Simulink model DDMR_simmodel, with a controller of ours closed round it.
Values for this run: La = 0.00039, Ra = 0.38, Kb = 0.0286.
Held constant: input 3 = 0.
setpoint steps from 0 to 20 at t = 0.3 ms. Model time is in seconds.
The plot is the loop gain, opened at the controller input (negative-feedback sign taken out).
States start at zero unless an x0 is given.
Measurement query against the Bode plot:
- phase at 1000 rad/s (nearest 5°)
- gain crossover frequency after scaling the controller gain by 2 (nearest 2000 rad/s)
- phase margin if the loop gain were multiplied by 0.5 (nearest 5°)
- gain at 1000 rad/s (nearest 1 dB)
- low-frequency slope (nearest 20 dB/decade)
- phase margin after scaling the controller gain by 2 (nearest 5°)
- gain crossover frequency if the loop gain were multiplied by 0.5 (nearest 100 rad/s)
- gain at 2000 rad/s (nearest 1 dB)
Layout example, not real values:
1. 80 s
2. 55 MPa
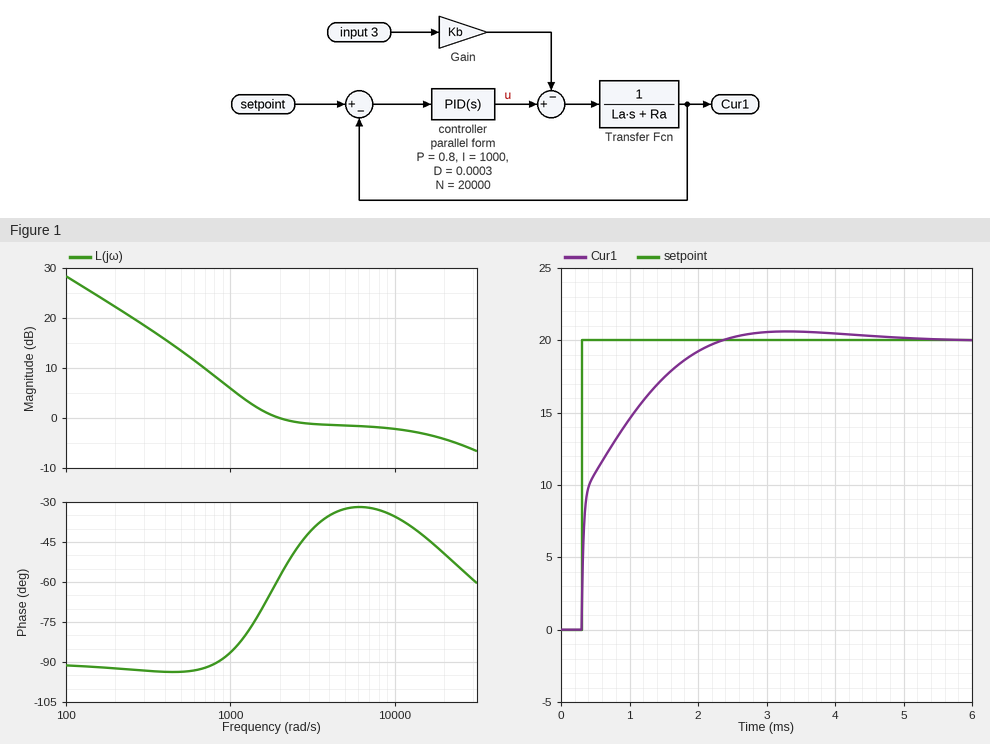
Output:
1. -85°
2. 28000 rad/s
3. 95°
4. 6 dB
5. -20 dB/decade
6. 120°
7. 1000 rad/s
8. 0 dB
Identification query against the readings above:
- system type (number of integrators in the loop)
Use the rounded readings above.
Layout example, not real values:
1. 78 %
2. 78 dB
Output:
1. 1
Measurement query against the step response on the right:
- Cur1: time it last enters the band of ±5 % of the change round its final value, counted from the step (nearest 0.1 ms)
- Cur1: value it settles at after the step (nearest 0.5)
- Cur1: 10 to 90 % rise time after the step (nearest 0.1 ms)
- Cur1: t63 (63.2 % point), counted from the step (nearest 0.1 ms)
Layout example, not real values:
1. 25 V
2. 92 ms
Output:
1. 1.6 ms
2. 20.0
3. 1.3 ms
4. 0.4 ms
